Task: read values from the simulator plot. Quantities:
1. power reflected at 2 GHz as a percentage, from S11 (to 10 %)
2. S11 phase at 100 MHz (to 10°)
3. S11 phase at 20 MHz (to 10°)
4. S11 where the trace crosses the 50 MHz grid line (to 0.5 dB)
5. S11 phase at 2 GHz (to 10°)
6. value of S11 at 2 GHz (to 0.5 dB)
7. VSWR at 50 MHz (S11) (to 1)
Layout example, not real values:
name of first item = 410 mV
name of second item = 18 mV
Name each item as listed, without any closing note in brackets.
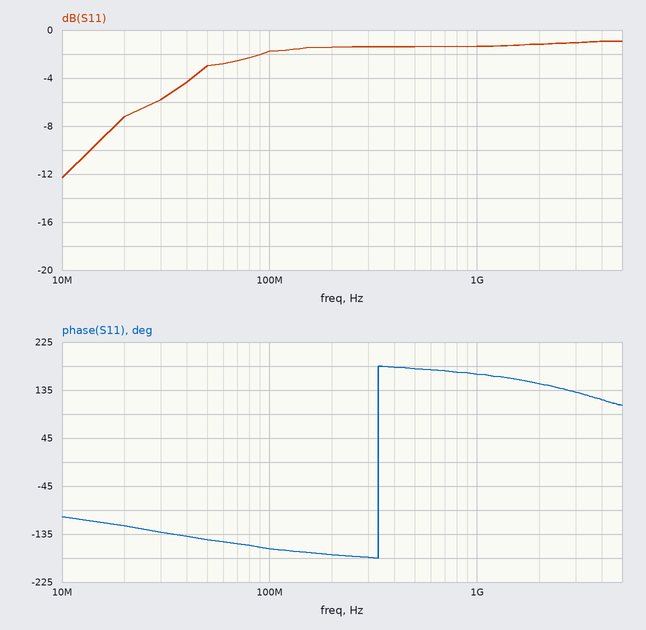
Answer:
power reflected at 2 GHz as a percentage, from S11 = 80 %
S11 phase at 100 MHz = -160°
S11 phase at 20 MHz = -120°
S11 where the trace crosses the 50 MHz grid line = -3.0 dB
S11 phase at 2 GHz = 150°
value of S11 at 2 GHz = -1.0 dB
VSWR at 50 MHz (S11) = 6
